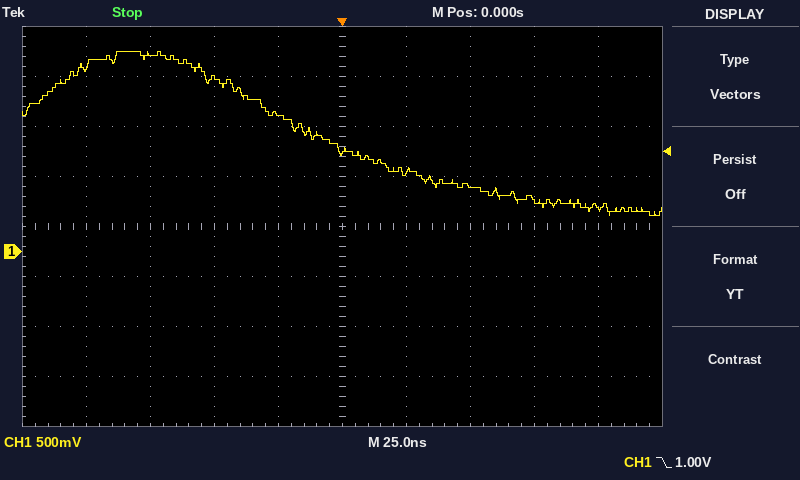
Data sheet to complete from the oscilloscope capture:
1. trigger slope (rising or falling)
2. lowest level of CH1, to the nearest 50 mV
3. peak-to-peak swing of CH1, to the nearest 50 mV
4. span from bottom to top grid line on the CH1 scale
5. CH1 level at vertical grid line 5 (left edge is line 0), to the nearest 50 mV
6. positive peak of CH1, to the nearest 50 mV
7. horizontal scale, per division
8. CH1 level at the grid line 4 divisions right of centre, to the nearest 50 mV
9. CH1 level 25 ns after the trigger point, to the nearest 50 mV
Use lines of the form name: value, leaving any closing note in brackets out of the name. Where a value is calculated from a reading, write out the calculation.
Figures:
trigger slope: falling
lowest level of CH1, to the nearest 50 mV: 350 mV
peak-to-peak swing of CH1, to the nearest 50 mV: 2.00 V − (350 mV) = 1.65 V
span from bottom to top grid line on the CH1 scale: 4 V
CH1 level at vertical grid line 5 (left edge is line 0), to the nearest 50 mV: 1.00 V
positive peak of CH1, to the nearest 50 mV: 2.00 V
horizontal scale, per division: 25 ns
CH1 level at the grid line 4 divisions right of centre, to the nearest 50 mV: 450 mV
CH1 level 25 ns after the trigger point, to the nearest 50 mV: 800 mV
